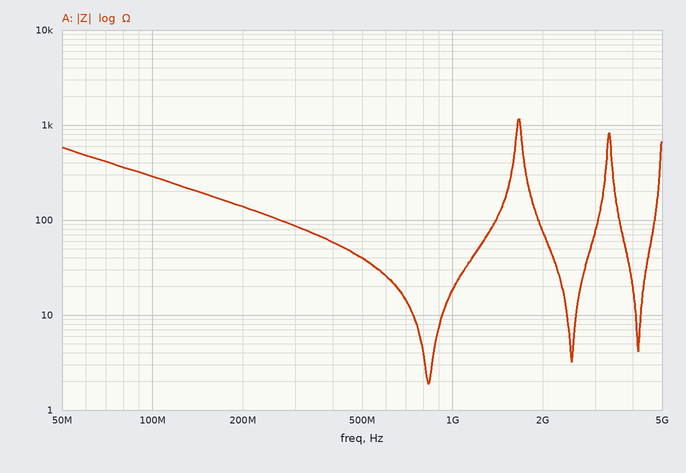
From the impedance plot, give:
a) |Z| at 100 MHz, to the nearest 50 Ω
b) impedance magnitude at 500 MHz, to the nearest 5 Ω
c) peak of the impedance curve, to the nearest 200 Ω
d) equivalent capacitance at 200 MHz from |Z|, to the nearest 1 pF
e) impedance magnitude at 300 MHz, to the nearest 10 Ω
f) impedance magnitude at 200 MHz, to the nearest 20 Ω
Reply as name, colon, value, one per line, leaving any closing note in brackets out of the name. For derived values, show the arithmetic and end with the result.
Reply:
|Z| at 100 MHz, to the nearest 50 Ω: 300 Ω
impedance magnitude at 500 MHz, to the nearest 5 Ω: 40 Ω
peak of the impedance curve, to the nearest 200 Ω: 1.2 kΩ
equivalent capacitance at 200 MHz from |Z|, to the nearest 1 pF: C = 1/(2π × 200 MHz × 140 Ω) ≈ 6 pF
impedance magnitude at 300 MHz, to the nearest 10 Ω: 90 Ω
impedance magnitude at 200 MHz, to the nearest 20 Ω: 140 Ω
